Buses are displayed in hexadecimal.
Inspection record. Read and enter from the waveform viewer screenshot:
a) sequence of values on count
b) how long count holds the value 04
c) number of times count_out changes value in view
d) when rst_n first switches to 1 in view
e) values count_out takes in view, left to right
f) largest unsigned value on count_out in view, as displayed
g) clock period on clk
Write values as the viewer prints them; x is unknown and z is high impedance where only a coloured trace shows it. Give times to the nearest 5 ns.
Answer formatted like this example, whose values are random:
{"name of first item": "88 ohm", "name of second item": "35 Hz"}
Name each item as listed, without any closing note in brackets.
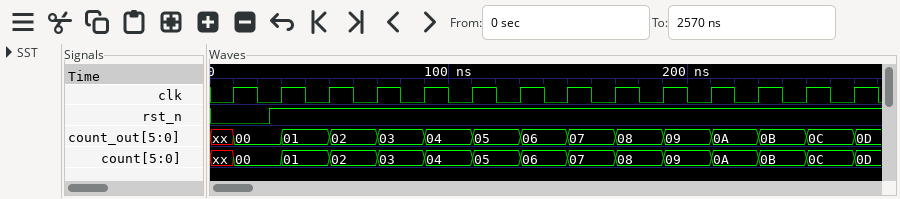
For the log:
{"sequence of values on count": "xx, 00, 01, 02, 03, 04, 05, 06, 07, 08, 09, 0A, 0B, 0C, 0D", "how long count holds the value 04": "20 ns", "number of times count_out changes value in view": "14", "when rst_n first switches to 1 in view": "25 ns", "values count_out takes in view, left to right": "xx, 00, 01, 02, 03, 04, 05, 06, 07, 08, 09, 0A, 0B, 0C, 0D", "largest unsigned value on count_out in view, as displayed": "0D", "clock period on clk": "20 ns"}
